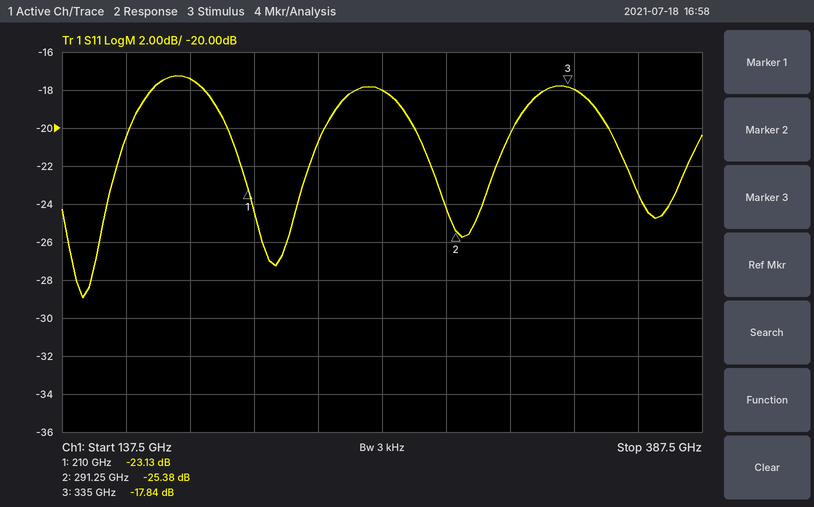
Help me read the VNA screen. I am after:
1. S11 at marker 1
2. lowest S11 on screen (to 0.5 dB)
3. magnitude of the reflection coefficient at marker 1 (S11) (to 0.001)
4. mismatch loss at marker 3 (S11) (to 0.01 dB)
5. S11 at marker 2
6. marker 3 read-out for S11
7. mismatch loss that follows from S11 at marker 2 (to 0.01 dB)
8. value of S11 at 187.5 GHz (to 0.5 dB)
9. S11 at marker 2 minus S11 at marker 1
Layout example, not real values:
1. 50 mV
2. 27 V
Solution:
1. -23.13 dB
2. -29.0 dB
3. 0.070
4. 0.07 dB
5. -25.38 dB
6. -17.84 dB
7. 0.01 dB
8. -17.5 dB
9. -2.25 dB
